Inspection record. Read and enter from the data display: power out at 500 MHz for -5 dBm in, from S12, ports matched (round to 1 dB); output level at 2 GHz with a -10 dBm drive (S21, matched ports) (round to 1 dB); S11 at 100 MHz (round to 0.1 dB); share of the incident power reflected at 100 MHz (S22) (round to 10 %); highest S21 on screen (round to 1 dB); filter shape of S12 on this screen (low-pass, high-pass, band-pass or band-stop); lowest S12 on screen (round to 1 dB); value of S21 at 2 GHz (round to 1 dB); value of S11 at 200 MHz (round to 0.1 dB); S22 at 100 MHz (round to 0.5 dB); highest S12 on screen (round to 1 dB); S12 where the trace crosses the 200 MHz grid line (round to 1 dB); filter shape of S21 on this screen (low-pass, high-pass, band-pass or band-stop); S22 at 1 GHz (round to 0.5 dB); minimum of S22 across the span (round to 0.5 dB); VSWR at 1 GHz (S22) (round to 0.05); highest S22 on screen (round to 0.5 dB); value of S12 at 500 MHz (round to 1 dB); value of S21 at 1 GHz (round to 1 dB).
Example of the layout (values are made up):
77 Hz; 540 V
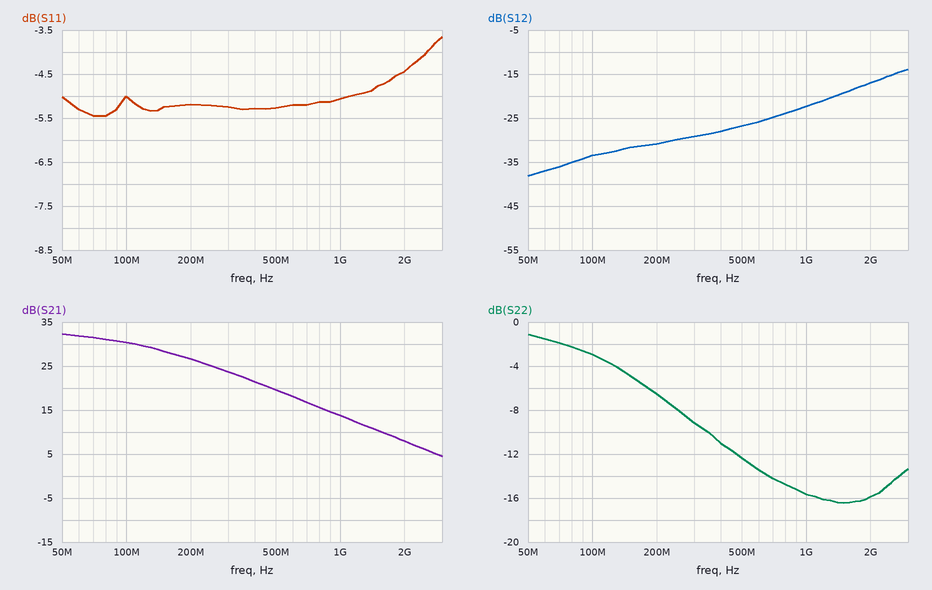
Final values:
-32 dBm; -2 dBm; -5.0 dB; 50 %; 32 dB; high-pass; -38 dB; 8 dB; -5.2 dB; -3.0 dB; -14 dB; -31 dB; low-pass; -15.5 dB; -16.5 dB; 1.40; -1.0 dB; -27 dB; 14 dB
